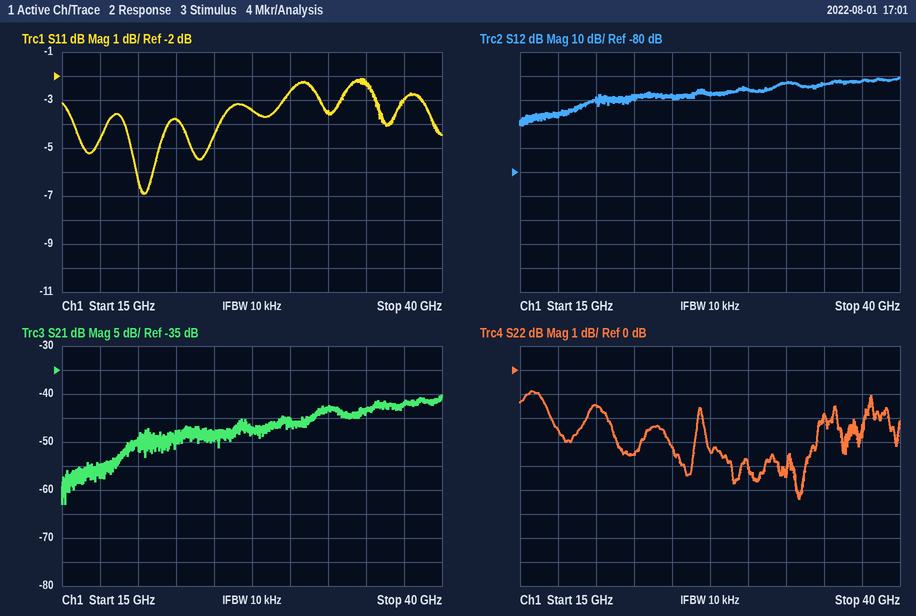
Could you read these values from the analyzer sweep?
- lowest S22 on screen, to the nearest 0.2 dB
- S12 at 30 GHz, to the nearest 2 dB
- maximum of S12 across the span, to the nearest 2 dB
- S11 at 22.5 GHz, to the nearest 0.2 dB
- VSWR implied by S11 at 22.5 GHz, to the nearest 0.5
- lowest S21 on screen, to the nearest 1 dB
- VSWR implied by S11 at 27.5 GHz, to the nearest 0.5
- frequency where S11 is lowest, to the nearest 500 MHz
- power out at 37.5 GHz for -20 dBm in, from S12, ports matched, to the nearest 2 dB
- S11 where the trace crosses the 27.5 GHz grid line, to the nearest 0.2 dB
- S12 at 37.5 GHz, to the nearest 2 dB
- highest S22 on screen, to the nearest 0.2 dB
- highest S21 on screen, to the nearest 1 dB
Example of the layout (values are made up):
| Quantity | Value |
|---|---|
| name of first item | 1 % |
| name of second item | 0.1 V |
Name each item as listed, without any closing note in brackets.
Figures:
| Quantity | Value |
|---|---|
| lowest S22 on screen, to the nearest 0.2 dB | -5.4 dB |
| S12 at 30 GHz, to the nearest 2 dB | -46 dB |
| maximum of S12 across the span, to the nearest 2 dB | -40 dB |
| S11 at 22.5 GHz, to the nearest 0.2 dB | -3.8 dB |
| VSWR implied by S11 at 22.5 GHz, to the nearest 0.5 | 4.5 |
| lowest S21 on screen, to the nearest 1 dB | -63 dB |
| VSWR implied by S11 at 27.5 GHz, to the nearest 0.5 | 5.0 |
| frequency where S11 is lowest, to the nearest 500 MHz | 20.5 GHz |
| power out at 37.5 GHz for -20 dBm in, from S12, ports matched, to the nearest 2 dB | -62 dBm |
| S11 where the trace crosses the 27.5 GHz grid line, to the nearest 0.2 dB | -3.4 dB |
| S12 at 37.5 GHz, to the nearest 2 dB | -42 dB |
| highest S22 on screen, to the nearest 0.2 dB | -0.8 dB |
| highest S21 on screen, to the nearest 1 dB | -40 dB |
